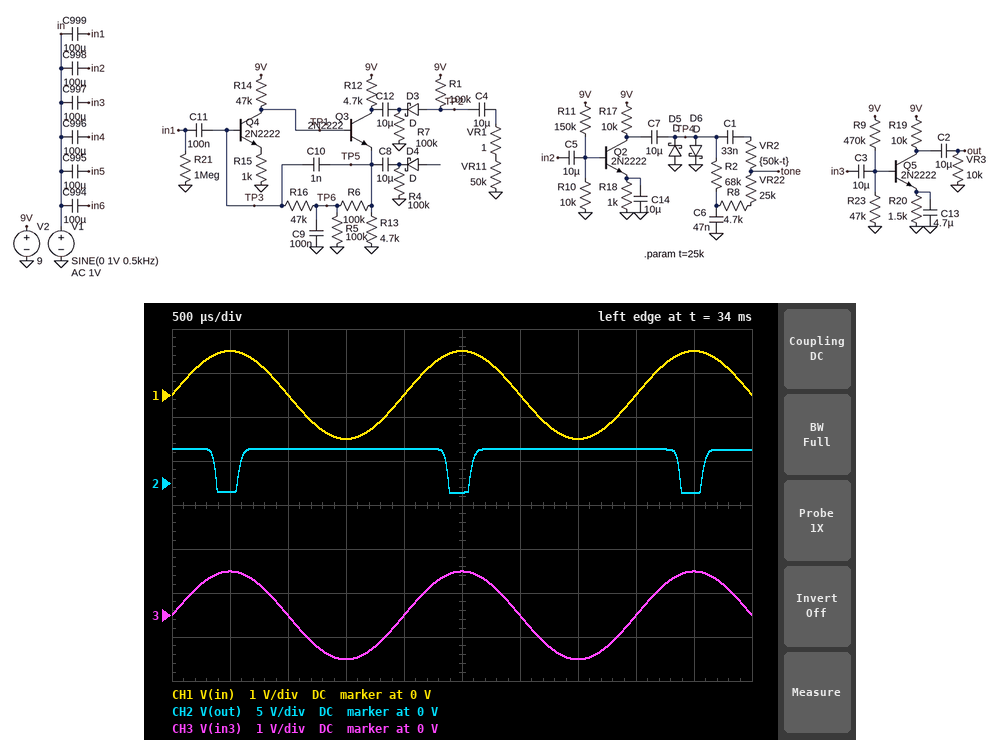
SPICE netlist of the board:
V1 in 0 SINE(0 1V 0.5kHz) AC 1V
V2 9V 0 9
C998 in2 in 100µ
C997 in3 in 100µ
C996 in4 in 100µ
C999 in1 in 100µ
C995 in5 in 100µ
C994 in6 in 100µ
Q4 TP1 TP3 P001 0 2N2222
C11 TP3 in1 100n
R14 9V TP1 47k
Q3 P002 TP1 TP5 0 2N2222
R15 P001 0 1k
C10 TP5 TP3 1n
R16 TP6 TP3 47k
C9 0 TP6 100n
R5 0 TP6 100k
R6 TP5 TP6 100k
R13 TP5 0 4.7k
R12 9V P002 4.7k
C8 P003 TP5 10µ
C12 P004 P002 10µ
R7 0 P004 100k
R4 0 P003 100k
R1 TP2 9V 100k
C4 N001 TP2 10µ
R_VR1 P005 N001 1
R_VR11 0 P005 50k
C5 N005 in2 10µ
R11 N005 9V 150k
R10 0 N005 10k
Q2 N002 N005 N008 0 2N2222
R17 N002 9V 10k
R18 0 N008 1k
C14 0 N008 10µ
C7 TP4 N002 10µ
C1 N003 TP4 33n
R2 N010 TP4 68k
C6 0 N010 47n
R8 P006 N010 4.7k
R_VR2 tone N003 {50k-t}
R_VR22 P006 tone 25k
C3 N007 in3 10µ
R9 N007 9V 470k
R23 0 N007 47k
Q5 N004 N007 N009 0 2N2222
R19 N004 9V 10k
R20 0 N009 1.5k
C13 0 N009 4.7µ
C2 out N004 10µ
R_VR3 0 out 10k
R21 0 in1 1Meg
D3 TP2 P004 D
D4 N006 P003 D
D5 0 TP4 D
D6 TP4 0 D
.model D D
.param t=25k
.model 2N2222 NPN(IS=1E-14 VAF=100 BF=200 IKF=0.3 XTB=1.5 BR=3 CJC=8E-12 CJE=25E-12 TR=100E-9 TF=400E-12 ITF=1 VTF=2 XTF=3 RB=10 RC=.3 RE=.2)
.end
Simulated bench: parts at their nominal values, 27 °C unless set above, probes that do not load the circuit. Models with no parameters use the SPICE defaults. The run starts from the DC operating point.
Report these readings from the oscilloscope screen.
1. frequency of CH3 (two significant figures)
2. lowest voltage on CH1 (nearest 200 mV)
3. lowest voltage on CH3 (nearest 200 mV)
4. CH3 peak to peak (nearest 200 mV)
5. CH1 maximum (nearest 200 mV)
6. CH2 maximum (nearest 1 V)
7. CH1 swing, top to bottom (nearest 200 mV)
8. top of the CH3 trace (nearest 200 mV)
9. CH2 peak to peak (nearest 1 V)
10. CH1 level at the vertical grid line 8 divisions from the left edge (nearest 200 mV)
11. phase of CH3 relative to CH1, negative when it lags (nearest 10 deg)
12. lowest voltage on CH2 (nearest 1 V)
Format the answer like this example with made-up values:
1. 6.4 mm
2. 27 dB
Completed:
1. 500 Hz
2. -1.0 V
3. -1.0 V
4. 2.0 V
5. 1.0 V
6. 4 V
7. 2.0 V
8. 1.0 V
9. 5 V
10. 0 V
11. 0 deg
12. -1 V
